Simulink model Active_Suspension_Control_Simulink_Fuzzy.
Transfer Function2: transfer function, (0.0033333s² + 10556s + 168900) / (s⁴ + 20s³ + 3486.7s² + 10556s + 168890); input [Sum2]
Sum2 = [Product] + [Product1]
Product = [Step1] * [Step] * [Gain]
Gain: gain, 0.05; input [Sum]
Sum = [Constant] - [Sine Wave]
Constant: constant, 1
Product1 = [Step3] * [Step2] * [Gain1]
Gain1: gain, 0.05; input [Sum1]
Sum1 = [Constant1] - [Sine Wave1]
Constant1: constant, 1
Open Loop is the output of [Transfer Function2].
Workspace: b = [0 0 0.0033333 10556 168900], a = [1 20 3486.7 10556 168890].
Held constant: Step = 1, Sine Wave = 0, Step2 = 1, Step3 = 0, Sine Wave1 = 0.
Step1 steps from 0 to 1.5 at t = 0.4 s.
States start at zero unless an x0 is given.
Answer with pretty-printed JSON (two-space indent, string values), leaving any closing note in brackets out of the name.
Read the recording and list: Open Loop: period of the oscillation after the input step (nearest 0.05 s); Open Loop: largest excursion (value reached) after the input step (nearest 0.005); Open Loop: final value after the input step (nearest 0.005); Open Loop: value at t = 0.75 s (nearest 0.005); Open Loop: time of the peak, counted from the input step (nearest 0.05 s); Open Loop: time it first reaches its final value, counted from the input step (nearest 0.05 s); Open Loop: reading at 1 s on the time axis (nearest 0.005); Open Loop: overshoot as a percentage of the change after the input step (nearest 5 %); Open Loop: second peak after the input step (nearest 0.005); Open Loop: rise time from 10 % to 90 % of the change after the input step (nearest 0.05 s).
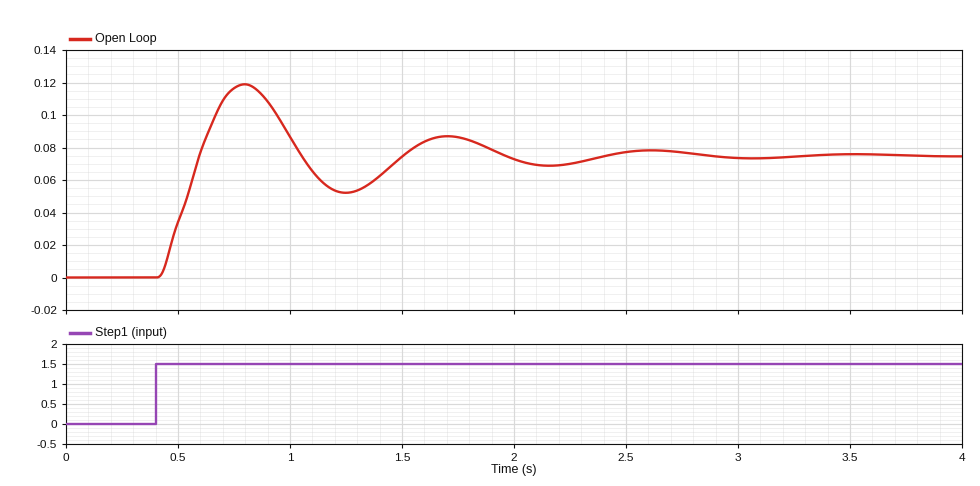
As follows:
{
  "Open Loop: period of the oscillation after the input step": "0.90 s",
  "Open Loop: largest excursion (value reached) after the input step": "0.120",
  "Open Loop: final value after the input step": "0.075",
  "Open Loop: value at t = 0.75 s": "0.115",
  "Open Loop: time of the peak, counted from the input step": "0.40 s",
  "Open Loop: time it first reaches its final value, counted from the input step": "0.20 s",
  "Open Loop: reading at 1 s on the time axis": "0.085",
  "Open Loop: overshoot as a percentage of the change after the input step": "60 %",
  "Open Loop: second peak after the input step": "0.085",
  "Open Loop: rise time from 10 % to 90 % of the change after the input step": "0.15 s"
}
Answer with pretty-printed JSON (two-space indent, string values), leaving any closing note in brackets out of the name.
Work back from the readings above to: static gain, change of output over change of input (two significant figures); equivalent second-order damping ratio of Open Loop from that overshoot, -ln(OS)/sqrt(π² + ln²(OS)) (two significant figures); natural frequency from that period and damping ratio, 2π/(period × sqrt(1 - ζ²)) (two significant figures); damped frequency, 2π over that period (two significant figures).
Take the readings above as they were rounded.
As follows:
{
  "static gain, change of output over change of input": "0.050",
  "equivalent second-order damping ratio of Open Loop from that overshoot, -ln(OS)/sqrt(π² + ln²(OS))": "0.16",
  "natural frequency from that period and damping ratio, 2π/(period × sqrt(1 - ζ²))": "7.1 rad/s",
  "damped frequency, 2π over that period": "7.0 rad/s"
}
